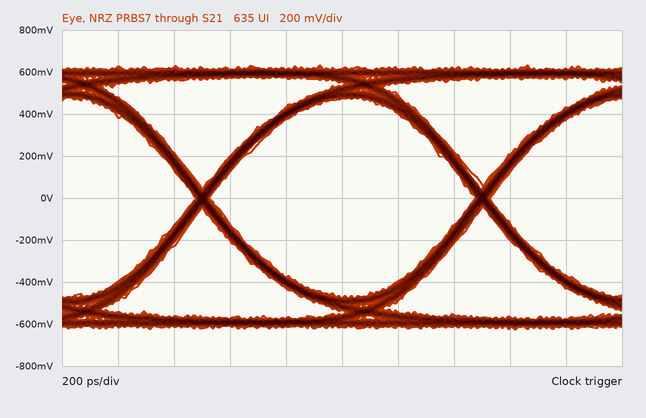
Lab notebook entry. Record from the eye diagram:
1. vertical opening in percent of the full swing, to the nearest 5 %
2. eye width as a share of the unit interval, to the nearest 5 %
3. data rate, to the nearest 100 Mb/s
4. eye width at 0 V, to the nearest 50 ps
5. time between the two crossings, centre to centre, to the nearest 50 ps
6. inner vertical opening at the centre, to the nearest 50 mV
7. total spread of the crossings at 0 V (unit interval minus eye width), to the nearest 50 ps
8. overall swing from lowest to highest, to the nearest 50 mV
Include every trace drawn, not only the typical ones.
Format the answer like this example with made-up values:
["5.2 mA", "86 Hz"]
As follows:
["75 %", "95 %", "1.0 Gb/s", "950 ps", "1.00 ns", "950 mV", "50 ps", "1.25 V"]
